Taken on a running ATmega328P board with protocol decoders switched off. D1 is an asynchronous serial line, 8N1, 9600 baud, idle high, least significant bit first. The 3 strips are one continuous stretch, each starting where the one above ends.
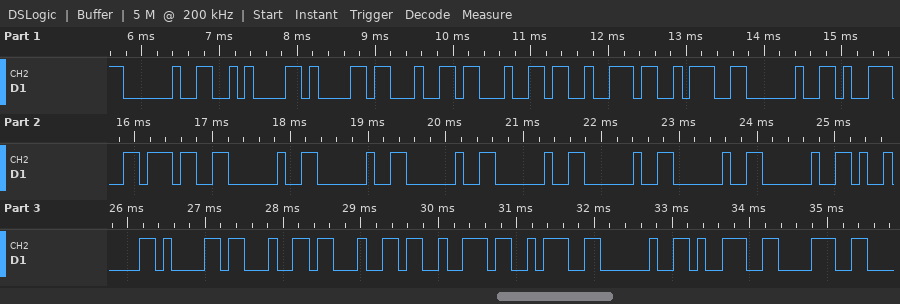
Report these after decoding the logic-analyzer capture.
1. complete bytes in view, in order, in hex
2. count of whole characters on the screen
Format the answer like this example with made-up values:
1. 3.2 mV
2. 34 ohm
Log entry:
1. 20 0A 61 64 64 72 3A 20 39 37 20 20 20 20 20 20 20 09 61 64 64 72 3A 20 39 38
2. 26
